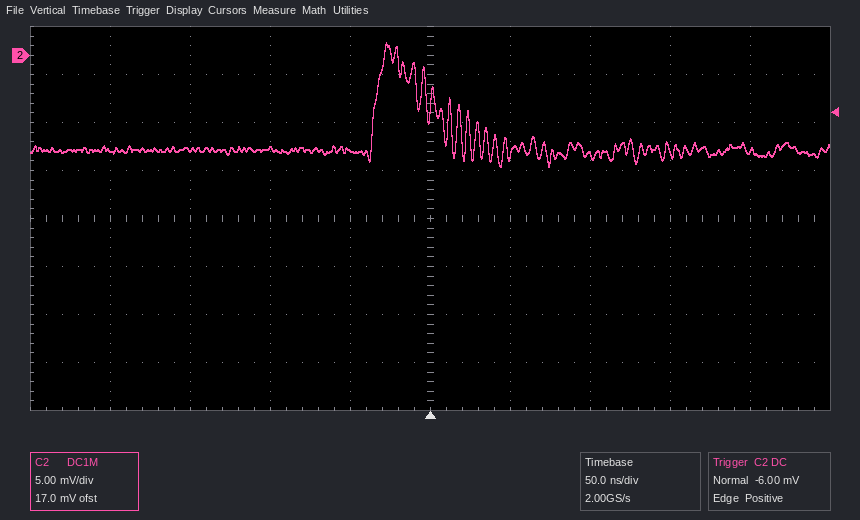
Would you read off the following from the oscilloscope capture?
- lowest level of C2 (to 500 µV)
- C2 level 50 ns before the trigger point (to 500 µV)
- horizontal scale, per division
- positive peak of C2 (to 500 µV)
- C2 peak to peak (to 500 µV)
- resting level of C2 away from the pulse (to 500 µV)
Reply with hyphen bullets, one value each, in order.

- -11.5 mV
- -10.0 mV
- 50 ns
- 1.5 mV
- 13.0 mV
- -10.0 mV
